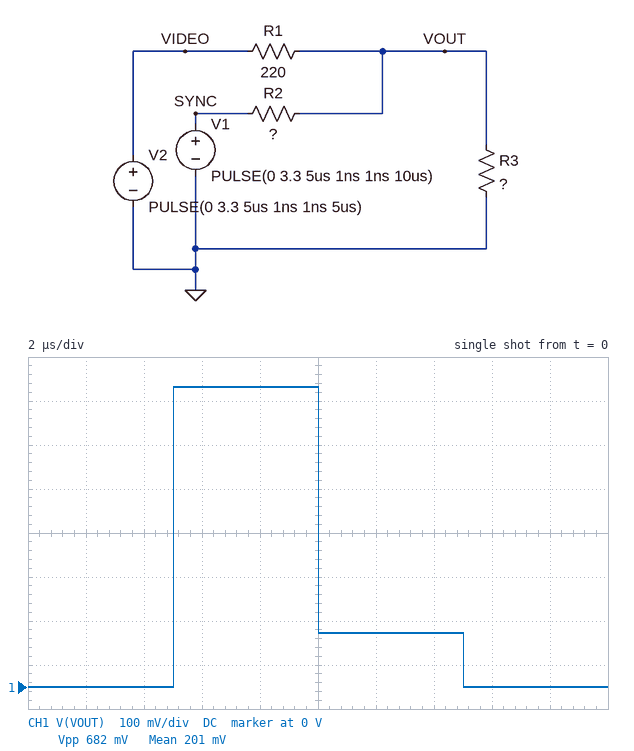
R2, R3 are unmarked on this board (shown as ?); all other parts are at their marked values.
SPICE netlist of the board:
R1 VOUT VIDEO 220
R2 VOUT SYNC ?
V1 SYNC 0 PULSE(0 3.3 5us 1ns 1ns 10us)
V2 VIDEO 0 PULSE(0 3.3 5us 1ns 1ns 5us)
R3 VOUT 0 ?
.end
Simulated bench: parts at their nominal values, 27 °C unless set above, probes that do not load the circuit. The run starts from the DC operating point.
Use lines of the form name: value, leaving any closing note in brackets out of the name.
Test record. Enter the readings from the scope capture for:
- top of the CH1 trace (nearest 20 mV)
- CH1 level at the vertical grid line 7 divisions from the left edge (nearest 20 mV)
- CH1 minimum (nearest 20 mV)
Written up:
top of the CH1 trace: 680 mV
CH1 level at the vertical grid line 7 divisions from the left edge: 120 mV
CH1 minimum: 0 V
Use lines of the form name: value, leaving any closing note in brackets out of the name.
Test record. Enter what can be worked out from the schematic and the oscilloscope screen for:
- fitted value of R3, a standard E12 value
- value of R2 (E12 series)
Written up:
fitted value of R3, a standard E12 value: 47 Ω
value of R2: 1 kΩ
